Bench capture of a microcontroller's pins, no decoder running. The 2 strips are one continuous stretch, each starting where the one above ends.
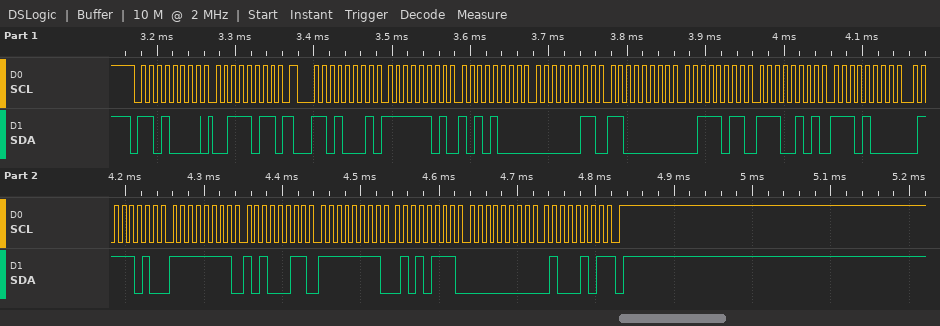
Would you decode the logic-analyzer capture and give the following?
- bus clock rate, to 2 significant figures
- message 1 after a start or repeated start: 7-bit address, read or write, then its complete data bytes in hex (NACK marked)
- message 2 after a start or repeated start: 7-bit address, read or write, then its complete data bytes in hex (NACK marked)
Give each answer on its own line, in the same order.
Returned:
100 kHz
0x68 write: 3B
0x68 read: FD A8 03 C0 3B E5 E8 7A FF A3 FF 57 00 45 NACK
